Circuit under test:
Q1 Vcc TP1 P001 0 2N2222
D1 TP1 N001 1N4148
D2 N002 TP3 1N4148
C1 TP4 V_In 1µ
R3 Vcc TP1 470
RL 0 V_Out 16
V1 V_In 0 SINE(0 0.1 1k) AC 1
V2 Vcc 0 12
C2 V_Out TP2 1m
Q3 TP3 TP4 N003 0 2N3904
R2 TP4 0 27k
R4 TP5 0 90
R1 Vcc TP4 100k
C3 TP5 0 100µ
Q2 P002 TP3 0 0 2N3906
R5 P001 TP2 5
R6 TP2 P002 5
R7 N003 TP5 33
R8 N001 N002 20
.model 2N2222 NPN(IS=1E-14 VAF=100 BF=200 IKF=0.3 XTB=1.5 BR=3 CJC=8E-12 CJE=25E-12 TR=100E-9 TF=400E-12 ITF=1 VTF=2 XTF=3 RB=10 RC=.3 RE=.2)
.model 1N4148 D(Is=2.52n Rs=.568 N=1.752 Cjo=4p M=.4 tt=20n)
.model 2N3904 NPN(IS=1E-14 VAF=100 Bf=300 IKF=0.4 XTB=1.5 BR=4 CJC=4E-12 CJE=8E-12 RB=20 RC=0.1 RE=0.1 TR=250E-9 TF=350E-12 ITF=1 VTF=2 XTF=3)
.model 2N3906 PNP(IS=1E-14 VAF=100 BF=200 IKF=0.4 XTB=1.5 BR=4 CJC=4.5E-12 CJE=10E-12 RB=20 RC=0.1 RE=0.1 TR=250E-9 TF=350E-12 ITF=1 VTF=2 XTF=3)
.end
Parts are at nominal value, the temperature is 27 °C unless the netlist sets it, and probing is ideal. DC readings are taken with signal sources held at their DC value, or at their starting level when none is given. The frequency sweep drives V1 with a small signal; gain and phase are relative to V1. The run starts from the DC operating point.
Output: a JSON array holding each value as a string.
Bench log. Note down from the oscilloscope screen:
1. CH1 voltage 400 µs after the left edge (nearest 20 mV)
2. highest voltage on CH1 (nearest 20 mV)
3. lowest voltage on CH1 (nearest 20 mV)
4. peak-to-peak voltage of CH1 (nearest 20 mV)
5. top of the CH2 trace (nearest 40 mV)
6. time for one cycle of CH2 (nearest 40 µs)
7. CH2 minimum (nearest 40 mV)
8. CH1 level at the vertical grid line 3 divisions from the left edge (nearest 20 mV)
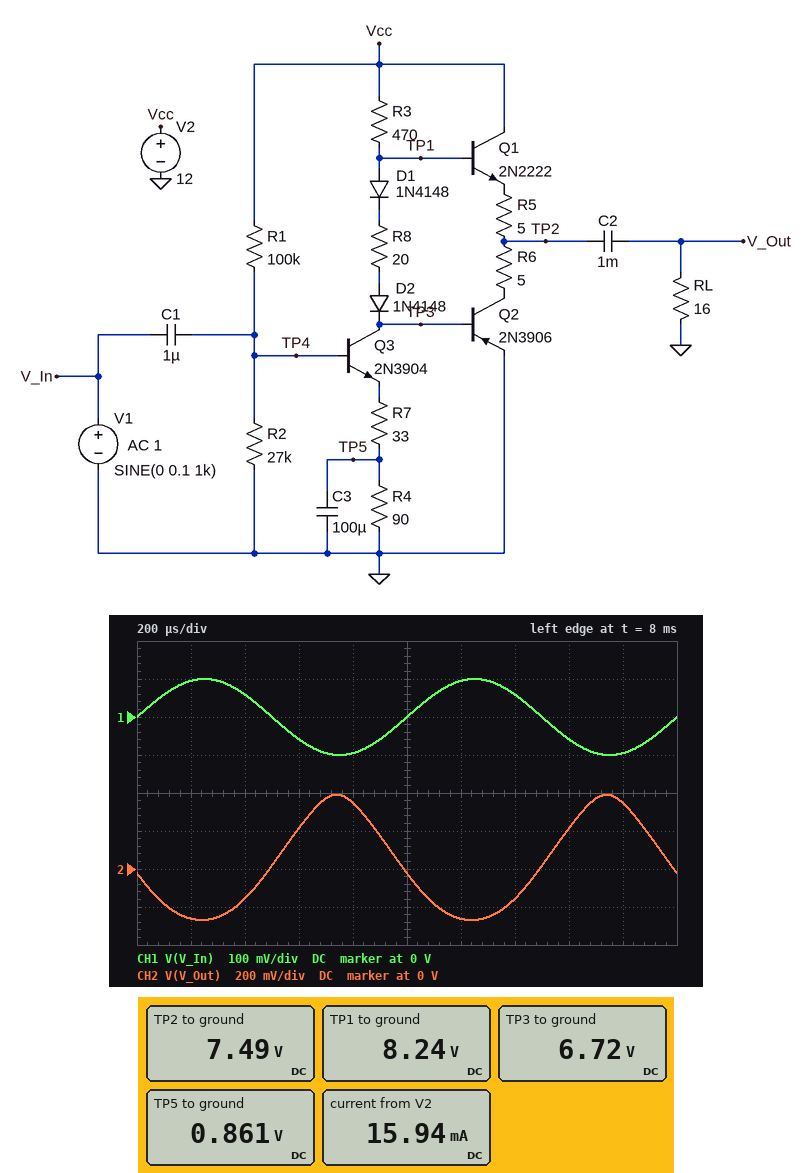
["60 mV", "100 mV", "-100 mV", "200 mV", "400 mV", "1.00 ms", "-280 mV", "-60 mV"]
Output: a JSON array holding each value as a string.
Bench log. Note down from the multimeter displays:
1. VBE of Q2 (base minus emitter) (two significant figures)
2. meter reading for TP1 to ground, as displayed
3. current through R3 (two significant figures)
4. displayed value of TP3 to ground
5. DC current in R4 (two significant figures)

["6.7 V", "8.24 V", "8.0 mA", "6.72 V", "9.6 mA"]
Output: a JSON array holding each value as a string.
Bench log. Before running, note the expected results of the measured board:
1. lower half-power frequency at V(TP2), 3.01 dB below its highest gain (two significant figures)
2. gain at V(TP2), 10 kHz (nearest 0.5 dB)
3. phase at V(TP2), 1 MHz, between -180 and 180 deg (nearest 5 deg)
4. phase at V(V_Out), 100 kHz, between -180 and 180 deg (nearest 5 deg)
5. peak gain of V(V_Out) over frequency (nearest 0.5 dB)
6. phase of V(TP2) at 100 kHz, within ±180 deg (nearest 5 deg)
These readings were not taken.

["70 Hz", "10.0 dB", "165 deg", "165 deg", "10.0 dB", "165 deg"]
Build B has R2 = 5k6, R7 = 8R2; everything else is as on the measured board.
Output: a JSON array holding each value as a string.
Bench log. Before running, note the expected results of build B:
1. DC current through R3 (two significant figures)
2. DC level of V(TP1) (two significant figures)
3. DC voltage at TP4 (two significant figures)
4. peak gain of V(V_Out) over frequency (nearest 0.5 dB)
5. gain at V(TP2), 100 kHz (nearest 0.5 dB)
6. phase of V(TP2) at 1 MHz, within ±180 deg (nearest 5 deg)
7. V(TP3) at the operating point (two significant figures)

["210 µA", "12 V", "630 mV", "-20.0 dB", "-30.0 dB", "-150 deg", "11 V"]
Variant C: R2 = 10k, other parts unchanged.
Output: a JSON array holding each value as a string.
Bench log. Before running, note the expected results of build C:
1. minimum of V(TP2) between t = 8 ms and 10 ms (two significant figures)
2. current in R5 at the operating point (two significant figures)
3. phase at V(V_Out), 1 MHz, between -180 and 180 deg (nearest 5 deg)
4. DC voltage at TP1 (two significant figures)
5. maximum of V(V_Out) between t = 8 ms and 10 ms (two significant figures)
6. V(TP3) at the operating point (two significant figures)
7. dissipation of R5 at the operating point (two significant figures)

["10 V", "840 µA", "150 deg", "11 V", "490 mV", "9.5 V", "3.5 µW"]
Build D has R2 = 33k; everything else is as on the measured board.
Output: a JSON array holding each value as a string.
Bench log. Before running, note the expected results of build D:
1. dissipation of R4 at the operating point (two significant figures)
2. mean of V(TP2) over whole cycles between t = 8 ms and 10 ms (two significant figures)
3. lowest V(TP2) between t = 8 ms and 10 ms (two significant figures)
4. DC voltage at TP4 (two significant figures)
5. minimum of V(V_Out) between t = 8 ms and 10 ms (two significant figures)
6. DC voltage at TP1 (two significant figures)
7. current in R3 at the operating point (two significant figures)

["11 mW", "7.0 V", "6.7 V", "2.1 V", "-280 mV", "7.7 V", "9.1 mA"]
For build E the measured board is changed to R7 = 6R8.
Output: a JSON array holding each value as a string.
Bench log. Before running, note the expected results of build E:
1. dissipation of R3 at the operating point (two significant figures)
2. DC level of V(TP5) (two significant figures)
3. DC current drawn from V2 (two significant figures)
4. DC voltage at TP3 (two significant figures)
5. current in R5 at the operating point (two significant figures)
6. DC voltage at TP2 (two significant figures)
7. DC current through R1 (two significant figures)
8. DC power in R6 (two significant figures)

["39 mW", "990 mV", "19 mA", "6.2 V", "9.6 mA", "7.0 V", "100 µA", "460 µW"]
